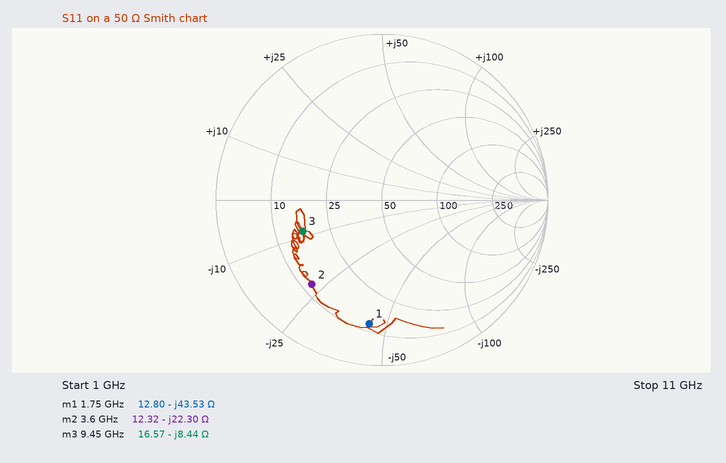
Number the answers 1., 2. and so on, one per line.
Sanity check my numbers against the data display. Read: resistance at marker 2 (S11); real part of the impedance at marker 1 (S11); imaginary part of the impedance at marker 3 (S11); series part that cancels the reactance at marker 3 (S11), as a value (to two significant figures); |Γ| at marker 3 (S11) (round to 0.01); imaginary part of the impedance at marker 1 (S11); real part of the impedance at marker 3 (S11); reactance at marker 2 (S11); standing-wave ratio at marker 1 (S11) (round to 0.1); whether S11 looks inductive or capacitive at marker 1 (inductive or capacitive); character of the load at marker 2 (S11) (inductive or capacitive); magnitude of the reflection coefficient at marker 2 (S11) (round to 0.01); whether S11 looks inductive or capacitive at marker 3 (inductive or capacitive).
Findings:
1. 12.32 Ω
2. 12.80 Ω
3. -8.44 Ω
4. 140 pH
5. 0.51
6. -43.53 Ω
7. 16.57 Ω
8. -22.30 Ω
9. 7.0
10. capacitive
11. capacitive
12. 0.66
13. capacitive
